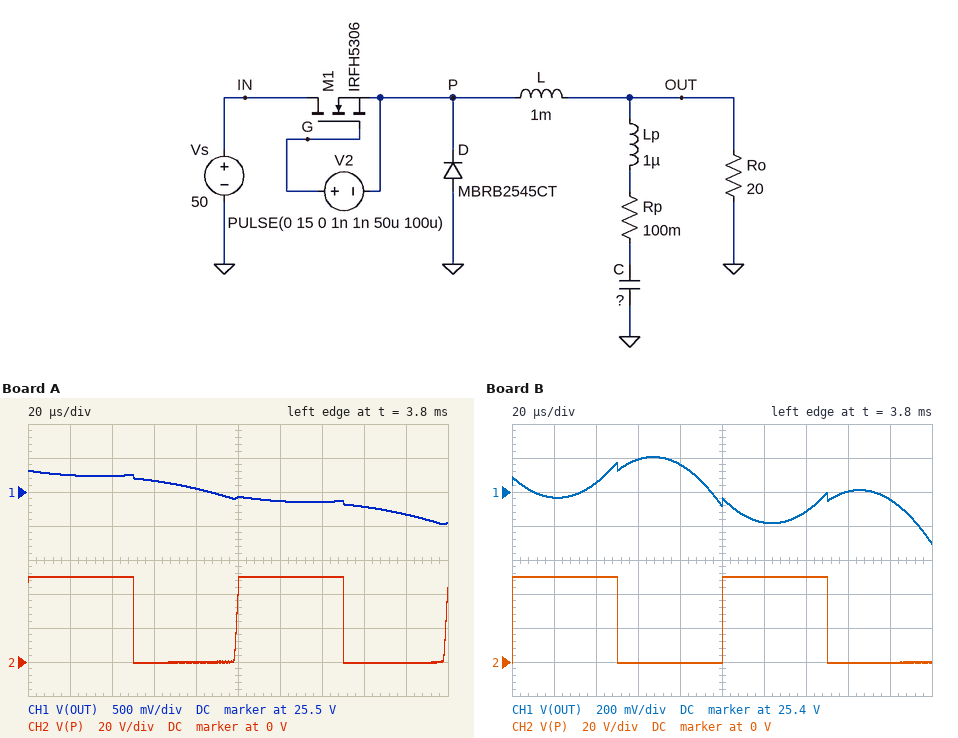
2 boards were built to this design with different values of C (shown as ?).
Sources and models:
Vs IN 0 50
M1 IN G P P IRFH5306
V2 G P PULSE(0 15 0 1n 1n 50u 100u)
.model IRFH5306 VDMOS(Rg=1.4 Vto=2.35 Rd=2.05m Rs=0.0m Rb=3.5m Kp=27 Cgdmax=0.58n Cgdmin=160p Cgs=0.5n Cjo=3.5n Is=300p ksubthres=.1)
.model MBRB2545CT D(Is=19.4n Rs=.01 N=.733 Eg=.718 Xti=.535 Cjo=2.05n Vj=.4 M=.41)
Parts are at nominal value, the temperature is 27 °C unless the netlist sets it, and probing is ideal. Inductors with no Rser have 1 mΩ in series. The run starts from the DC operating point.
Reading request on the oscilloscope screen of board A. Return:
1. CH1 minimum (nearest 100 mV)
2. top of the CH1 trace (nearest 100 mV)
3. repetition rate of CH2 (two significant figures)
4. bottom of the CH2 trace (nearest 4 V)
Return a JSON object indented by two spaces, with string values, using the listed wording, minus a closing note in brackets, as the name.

{
  "CH1 minimum": "25.0 V",
  "top of the CH1 trace": "25.8 V",
  "repetition rate of CH2": "10 kHz",
  "bottom of the CH2 trace": "0 V"
}
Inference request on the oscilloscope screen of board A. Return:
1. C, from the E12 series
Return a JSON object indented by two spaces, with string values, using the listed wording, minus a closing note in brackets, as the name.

{
  "C, from the E12 series": "180 µF"
}
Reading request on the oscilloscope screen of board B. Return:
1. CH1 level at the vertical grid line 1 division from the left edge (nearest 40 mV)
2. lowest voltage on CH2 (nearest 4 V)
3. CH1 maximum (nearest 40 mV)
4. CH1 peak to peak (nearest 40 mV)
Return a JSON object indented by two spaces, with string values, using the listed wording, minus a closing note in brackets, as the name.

{
  "CH1 level at the vertical grid line 1 division from the left edge": "25.36 V",
  "lowest voltage on CH2": "0 V",
  "CH1 maximum": "25.60 V",
  "CH1 peak to peak": "520 mV"
}
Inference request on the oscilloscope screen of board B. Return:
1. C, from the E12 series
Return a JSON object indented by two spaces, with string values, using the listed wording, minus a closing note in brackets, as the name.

{
  "C, from the E12 series": "47 µF"
}
